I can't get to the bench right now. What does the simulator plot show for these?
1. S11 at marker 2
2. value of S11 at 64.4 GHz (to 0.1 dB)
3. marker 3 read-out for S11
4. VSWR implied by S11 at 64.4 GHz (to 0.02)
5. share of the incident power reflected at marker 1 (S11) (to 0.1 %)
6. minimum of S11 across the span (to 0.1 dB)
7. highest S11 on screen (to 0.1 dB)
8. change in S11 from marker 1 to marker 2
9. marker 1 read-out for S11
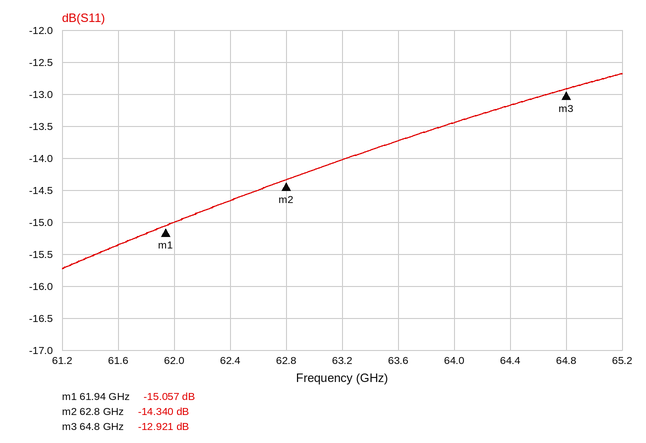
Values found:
-14.340 dB
-13.2 dB
-12.921 dB
1.56
3.1 %
-15.7 dB
-12.7 dB
0.717 dB
-15.057 dB
